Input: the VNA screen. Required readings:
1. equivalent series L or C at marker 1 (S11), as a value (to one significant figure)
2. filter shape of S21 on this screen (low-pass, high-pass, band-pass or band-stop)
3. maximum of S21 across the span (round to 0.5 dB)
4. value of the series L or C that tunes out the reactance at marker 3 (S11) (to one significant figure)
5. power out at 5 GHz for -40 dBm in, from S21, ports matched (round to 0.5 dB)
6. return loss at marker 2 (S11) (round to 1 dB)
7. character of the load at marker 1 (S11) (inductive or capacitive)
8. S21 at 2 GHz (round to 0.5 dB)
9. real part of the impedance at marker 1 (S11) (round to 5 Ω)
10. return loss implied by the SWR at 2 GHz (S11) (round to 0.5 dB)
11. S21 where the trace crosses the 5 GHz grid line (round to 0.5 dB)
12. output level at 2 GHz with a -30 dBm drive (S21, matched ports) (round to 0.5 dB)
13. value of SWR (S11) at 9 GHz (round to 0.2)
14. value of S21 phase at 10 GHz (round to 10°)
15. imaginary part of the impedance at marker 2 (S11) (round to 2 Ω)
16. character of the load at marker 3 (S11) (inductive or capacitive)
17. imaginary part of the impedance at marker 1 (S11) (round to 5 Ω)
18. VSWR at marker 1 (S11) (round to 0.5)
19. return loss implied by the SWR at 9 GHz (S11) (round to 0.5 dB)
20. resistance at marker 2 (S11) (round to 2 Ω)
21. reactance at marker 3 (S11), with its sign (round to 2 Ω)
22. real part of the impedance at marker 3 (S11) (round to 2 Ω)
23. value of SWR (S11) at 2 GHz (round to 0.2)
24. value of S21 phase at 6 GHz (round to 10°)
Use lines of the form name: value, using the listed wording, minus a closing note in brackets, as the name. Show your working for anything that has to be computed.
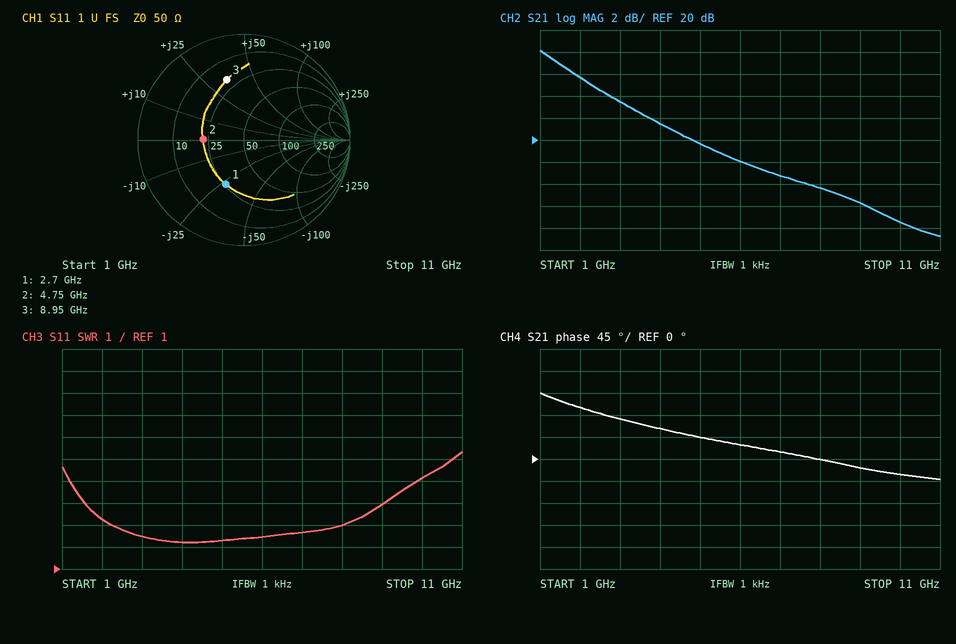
equivalent series L or C at marker 1 (S11), as a value: C = 1/(2π × 2.7 GHz × 25 Ω) ≈ 2 pF
filter shape of S21 on this screen: low-pass
maximum of S21 across the span: 28.0 dB
value of the series L or C that tunes out the reactance at marker 3 (S11): C = 1/(2π × 8.95 GHz × 34 Ω) ≈ 523 fF, so 500 fF to one significant figure
power out at 5 GHz for -40 dBm in, from S21, ports matched: -40 dBm + (19.5 dB) = -20.5 dBm
return loss at marker 2 (S11): 8 dB
character of the load at marker 1 (S11): capacitive
S21 at 2 GHz: 25.5 dB
real part of the impedance at marker 1 (S11): 25 Ω
return loss implied by the SWR at 2 GHz (S11): −20 log10((3.2 − 1)/(3.2 + 1)) ≈ 5.62 dB, so 5.5 dB to the nearest 0.5 dB
S21 where the trace crosses the 5 GHz grid line: 19.5 dB
output level at 2 GHz with a -30 dBm drive (S21, matched ports): -30 dBm + (25.5 dB) = -4.5 dBm
value of SWR (S11) at 9 GHz: 4.0
value of S21 phase at 10 GHz: -30°
imaginary part of the impedance at marker 2 (S11): 0 Ω
character of the load at marker 3 (S11): inductive
imaginary part of the impedance at marker 1 (S11): -25 Ω
VSWR at marker 1 (S11): 2.5
return loss implied by the SWR at 9 GHz (S11): −20 log10((4 − 1)/(4 + 1)) ≈ 4.44 dB, so 4.5 dB to the nearest 0.5 dB
resistance at marker 2 (S11): 22 Ω
reactance at marker 3 (S11), with its sign: +34 Ω
real part of the impedance at marker 3 (S11): 20 Ω
value of SWR (S11) at 2 GHz: 3.2
value of S21 phase at 6 GHz: 30°
